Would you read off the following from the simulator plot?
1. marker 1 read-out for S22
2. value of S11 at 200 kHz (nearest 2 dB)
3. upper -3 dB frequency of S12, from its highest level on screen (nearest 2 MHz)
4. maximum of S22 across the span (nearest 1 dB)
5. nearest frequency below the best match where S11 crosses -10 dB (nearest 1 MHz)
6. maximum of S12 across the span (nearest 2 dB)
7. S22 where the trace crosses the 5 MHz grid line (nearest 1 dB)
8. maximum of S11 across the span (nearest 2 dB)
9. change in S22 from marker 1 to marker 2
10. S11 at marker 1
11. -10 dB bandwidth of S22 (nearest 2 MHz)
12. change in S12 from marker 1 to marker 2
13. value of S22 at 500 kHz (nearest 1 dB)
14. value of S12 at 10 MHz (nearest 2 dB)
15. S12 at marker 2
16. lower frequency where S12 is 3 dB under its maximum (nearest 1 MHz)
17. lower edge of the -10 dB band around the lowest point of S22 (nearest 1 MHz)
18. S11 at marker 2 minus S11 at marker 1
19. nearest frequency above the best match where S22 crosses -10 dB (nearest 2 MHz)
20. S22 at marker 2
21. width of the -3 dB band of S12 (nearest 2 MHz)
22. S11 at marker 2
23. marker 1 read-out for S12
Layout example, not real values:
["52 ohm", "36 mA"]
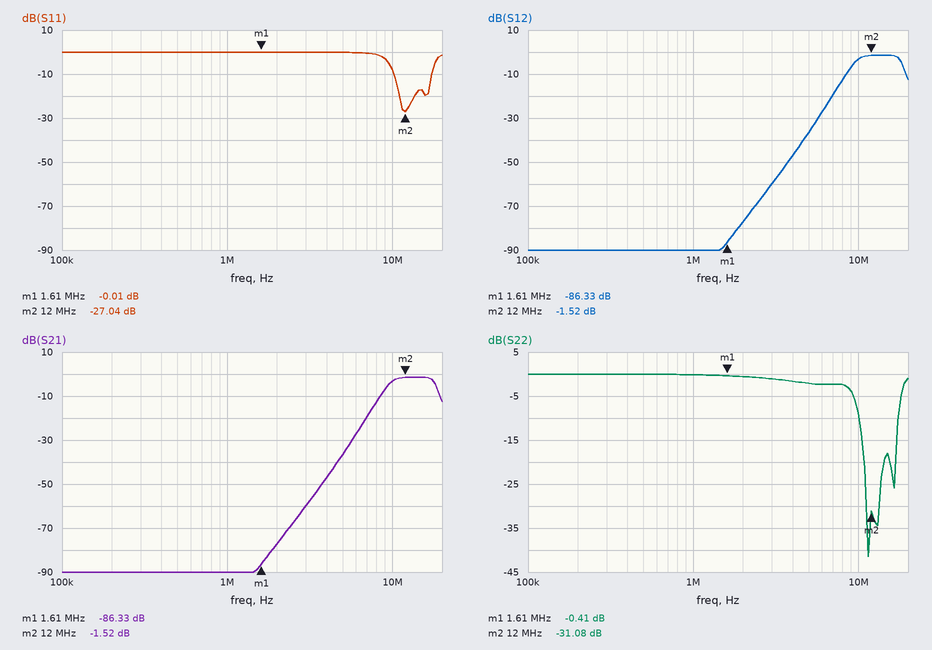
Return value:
["-0.41 dB", "0 dB", "18 MHz", "0 dB", "10 MHz", "-2 dB", "-2 dB", "0 dB", "-30.67 dB", "-0.01 dB", "8 MHz", "84.81 dB", "0 dB", "-4 dB", "-1.52 dB", "10 MHz", "10 MHz", "-27.03 dB", "18 MHz", "-31.08 dB", "8 MHz", "-27.04 dB", "-86.33 dB"]
